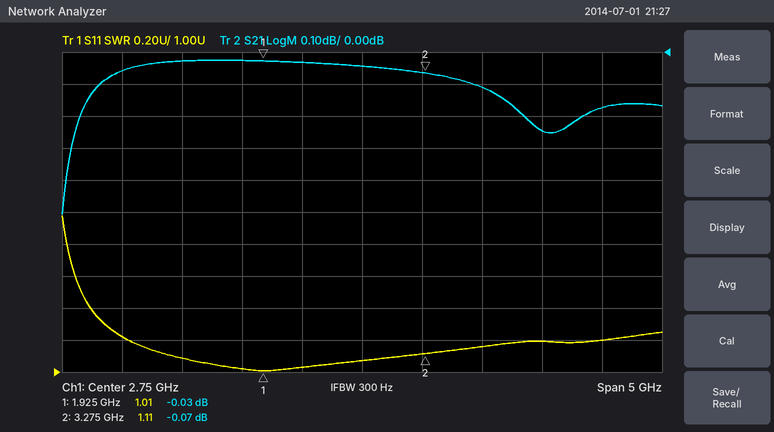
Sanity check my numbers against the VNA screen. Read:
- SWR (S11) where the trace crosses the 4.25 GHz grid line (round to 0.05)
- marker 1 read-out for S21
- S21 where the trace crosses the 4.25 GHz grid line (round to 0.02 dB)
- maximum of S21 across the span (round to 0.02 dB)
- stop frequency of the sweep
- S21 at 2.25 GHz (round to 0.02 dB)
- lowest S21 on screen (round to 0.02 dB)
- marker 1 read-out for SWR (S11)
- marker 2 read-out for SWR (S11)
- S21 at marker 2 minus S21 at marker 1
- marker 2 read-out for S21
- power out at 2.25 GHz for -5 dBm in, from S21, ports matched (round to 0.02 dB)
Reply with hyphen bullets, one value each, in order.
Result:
- 1.20
- -0.03 dB
- -0.24 dB
- -0.02 dB
- 5.25 GHz
- -0.04 dB
- -0.50 dB
- 1.01
- 1.11
- -0.04 dB
- -0.07 dB
- -5.04 dBm
